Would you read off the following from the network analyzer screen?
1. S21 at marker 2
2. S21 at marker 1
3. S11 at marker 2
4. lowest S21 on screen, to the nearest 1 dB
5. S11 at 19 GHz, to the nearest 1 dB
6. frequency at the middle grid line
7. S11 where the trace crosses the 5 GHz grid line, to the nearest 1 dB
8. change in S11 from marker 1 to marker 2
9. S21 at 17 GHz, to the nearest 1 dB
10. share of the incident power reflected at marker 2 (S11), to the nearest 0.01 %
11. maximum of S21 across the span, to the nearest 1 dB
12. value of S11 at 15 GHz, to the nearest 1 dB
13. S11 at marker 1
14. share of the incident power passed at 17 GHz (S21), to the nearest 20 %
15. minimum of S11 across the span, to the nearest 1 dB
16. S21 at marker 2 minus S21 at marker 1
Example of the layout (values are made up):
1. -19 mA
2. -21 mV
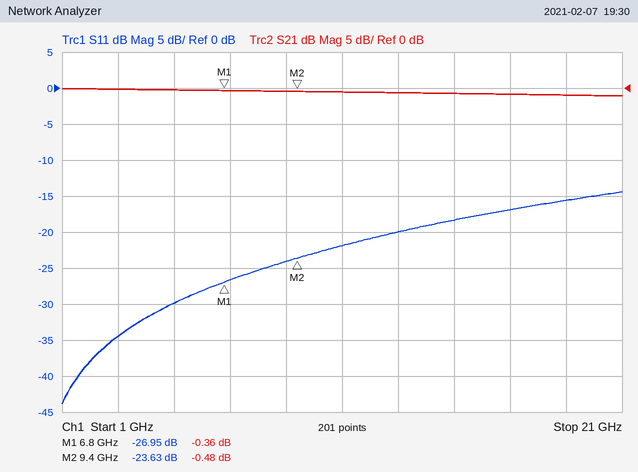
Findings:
1. -0.48 dB
2. -0.36 dB
3. -23.63 dB
4. -1 dB
5. -16 dB
6. 11 GHz
7. -30 dB
8. 3.32 dB
9. -1 dB
10. 0.43 %
11. 0 dB
12. -18 dB
13. -26.95 dB
14. 80 %
15. -44 dB
16. -0.12 dB
